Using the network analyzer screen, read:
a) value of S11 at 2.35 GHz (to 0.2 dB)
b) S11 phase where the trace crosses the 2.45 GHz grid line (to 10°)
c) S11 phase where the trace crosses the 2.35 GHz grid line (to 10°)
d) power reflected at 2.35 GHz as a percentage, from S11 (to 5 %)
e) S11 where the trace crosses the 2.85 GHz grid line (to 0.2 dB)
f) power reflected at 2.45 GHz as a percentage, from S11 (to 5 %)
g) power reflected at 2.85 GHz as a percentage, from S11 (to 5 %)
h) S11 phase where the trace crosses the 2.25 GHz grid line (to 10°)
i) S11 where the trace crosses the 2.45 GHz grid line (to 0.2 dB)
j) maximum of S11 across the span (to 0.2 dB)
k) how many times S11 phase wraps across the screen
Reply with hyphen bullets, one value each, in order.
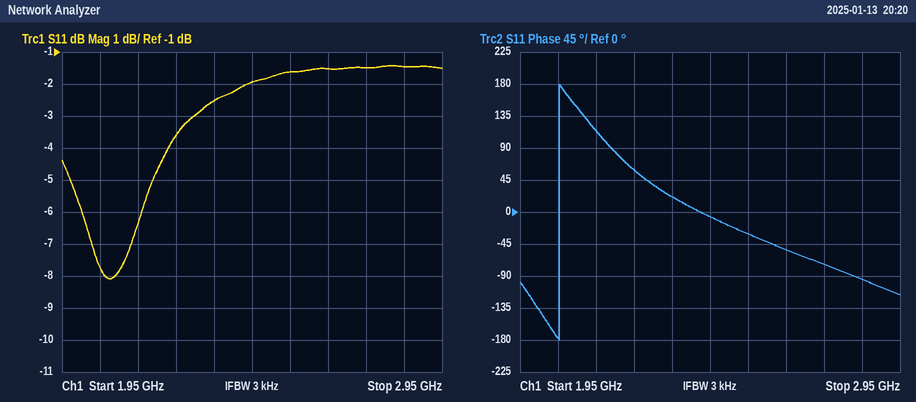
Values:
- -2.6 dB
- -10°
- 20°
- 55 %
- -1.4 dB
- 65 %
- 70 %
- 60°
- -2.0 dB
- -1.4 dB
- 1
